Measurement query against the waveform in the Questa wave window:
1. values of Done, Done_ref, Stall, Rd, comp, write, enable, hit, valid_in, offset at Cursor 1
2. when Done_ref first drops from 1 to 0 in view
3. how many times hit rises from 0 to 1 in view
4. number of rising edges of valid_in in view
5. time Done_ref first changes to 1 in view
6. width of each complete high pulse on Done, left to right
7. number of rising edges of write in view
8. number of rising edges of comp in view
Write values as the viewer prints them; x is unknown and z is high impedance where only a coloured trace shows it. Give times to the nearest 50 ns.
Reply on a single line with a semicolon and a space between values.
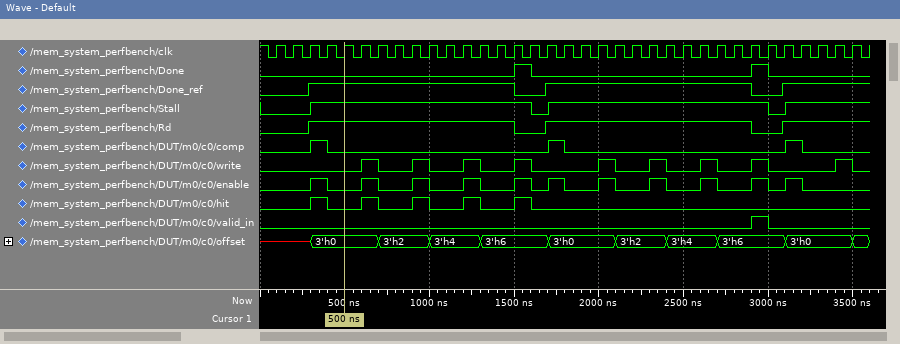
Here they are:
Done=0, Done_ref=1, Stall=1, Rd=1, comp=0, write=0, enable=0, hit=0, valid_in=0, offset=3'h0; 1500 ns; 5; 1; 300 ns; 100 ns, 100 ns; 9; 3
